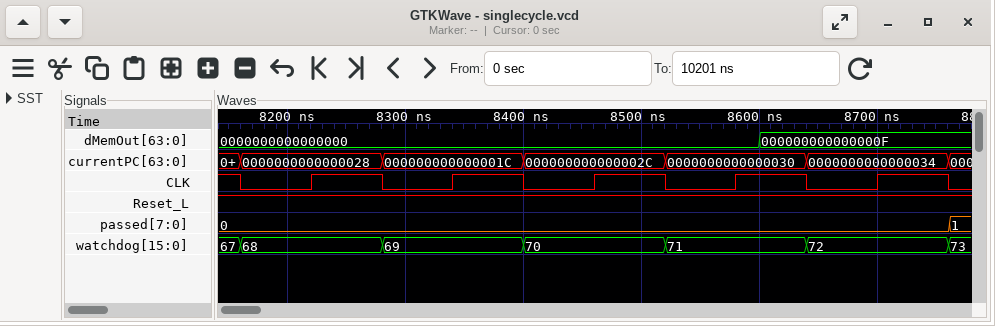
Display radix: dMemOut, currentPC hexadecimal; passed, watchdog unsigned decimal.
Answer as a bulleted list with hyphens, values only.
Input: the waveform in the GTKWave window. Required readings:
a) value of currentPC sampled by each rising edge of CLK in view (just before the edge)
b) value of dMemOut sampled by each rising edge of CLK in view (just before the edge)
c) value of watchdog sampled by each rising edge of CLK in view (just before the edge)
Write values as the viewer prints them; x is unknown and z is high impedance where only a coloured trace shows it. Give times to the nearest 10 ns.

- 0000000000000028, 000000000000001C, 000000000000002C, 0000000000000030, 0000000000000034
- 0000000000000000, 0000000000000000, 0000000000000000, 0000000000000000, 000000000000000F
- 68, 69, 70, 71, 72
